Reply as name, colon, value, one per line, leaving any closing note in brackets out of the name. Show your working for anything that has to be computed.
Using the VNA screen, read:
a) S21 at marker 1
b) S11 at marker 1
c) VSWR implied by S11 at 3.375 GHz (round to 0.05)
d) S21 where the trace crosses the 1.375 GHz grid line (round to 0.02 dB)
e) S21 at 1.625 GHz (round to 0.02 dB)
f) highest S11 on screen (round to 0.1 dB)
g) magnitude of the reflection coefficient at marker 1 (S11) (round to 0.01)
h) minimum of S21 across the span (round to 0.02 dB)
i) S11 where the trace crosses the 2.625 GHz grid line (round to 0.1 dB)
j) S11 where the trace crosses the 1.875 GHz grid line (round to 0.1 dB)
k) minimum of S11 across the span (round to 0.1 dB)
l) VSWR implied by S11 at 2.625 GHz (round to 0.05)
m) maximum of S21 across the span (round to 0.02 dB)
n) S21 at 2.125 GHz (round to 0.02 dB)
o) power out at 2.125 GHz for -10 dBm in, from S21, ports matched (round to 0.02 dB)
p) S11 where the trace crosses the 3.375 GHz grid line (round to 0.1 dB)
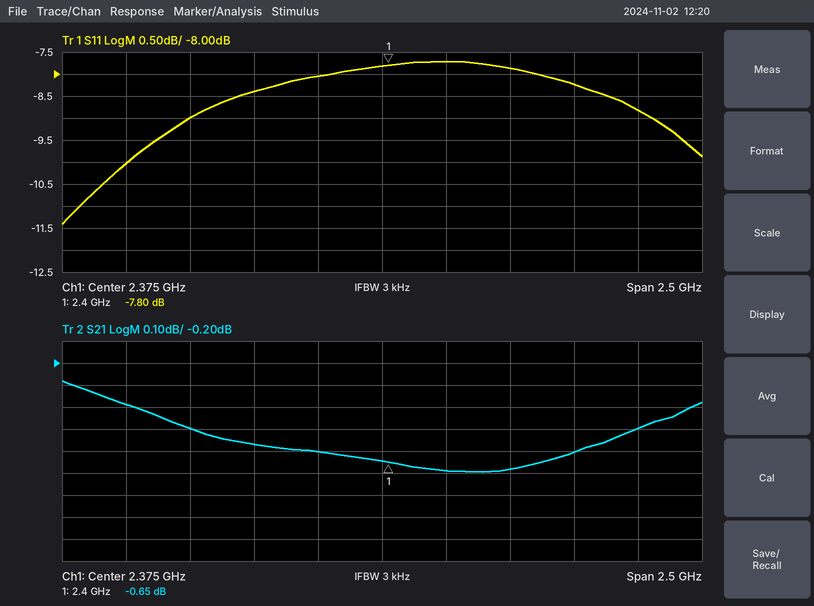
S21 at marker 1: -0.65 dB
S11 at marker 1: -7.80 dB
VSWR implied by S11 at 3.375 GHz: |Γ| = 10^(-8.8/20) = 0.3631; VSWR = (1 + 0.3631)/(1 − 0.3631) ≈ 2.14, so 2.15 to the nearest 0.05
S21 where the trace crosses the 1.375 GHz grid line: -0.38 dB
S21 at 1.625 GHz: -0.50 dB
highest S11 on screen: -7.7 dB
magnitude of the reflection coefficient at marker 1 (S11): 10^(-7.8/20) ≈ 0.41
minimum of S21 across the span: -0.70 dB
S11 where the trace crosses the 2.625 GHz grid line: -7.7 dB
S11 where the trace crosses the 1.875 GHz grid line: -8.4 dB
minimum of S11 across the span: -11.4 dB
VSWR implied by S11 at 2.625 GHz: |Γ| = 10^(-7.7/20) = 0.4121; VSWR = (1 + 0.4121)/(1 − 0.4121) ≈ 2.40
maximum of S21 across the span: -0.28 dB
S21 at 2.125 GHz: -0.60 dB
power out at 2.125 GHz for -10 dBm in, from S21, ports matched: -10 dBm + (-0.60 dB) = -10.60 dBm
S11 where the trace crosses the 3.375 GHz grid line: -8.8 dB
